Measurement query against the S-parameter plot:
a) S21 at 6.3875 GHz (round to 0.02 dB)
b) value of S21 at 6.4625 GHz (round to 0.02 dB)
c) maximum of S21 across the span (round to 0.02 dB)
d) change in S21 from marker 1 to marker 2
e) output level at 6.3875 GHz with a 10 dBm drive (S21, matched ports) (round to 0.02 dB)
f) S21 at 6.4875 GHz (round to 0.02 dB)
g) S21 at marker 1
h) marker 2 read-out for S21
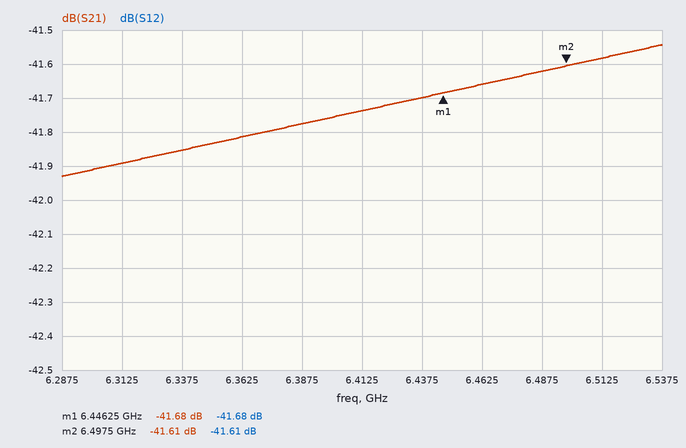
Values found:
-41.78 dB
-41.66 dB
-41.54 dB
0.07 dB
-31.78 dBm
-41.62 dB
-41.68 dB
-41.61 dB
